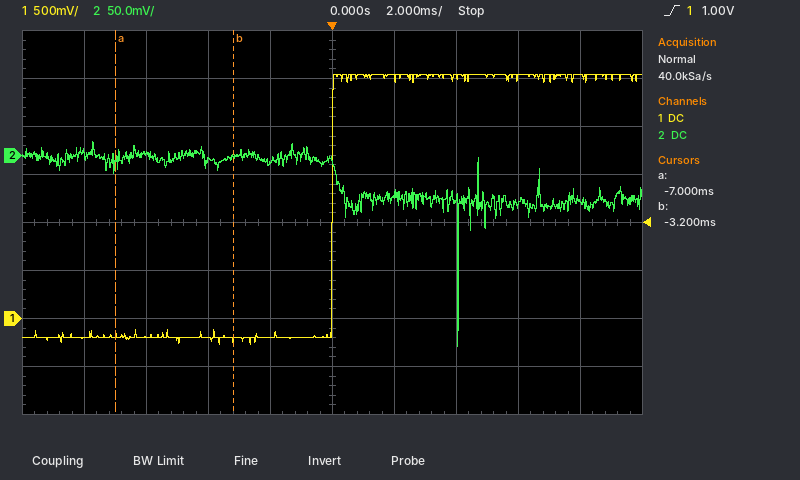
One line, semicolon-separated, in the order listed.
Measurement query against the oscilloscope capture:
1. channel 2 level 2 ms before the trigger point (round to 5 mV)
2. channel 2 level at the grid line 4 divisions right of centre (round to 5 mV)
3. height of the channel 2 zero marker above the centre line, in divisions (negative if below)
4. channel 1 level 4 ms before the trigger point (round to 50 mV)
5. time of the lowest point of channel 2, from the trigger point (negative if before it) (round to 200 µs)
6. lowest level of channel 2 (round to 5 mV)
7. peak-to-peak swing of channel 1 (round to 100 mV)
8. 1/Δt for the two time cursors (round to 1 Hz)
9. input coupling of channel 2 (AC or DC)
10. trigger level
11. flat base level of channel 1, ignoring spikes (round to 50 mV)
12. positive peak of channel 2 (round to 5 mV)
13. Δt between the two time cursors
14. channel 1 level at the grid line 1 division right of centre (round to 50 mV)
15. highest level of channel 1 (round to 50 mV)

-5 mV; -45 mV; +1.4 div; -200 mV; +4.0 ms; -200 mV; 2.80 V; 263 Hz; DC; 1.00 V; -200 mV; 15 mV; 3.8 ms; 2.50 V; 2.55 V
